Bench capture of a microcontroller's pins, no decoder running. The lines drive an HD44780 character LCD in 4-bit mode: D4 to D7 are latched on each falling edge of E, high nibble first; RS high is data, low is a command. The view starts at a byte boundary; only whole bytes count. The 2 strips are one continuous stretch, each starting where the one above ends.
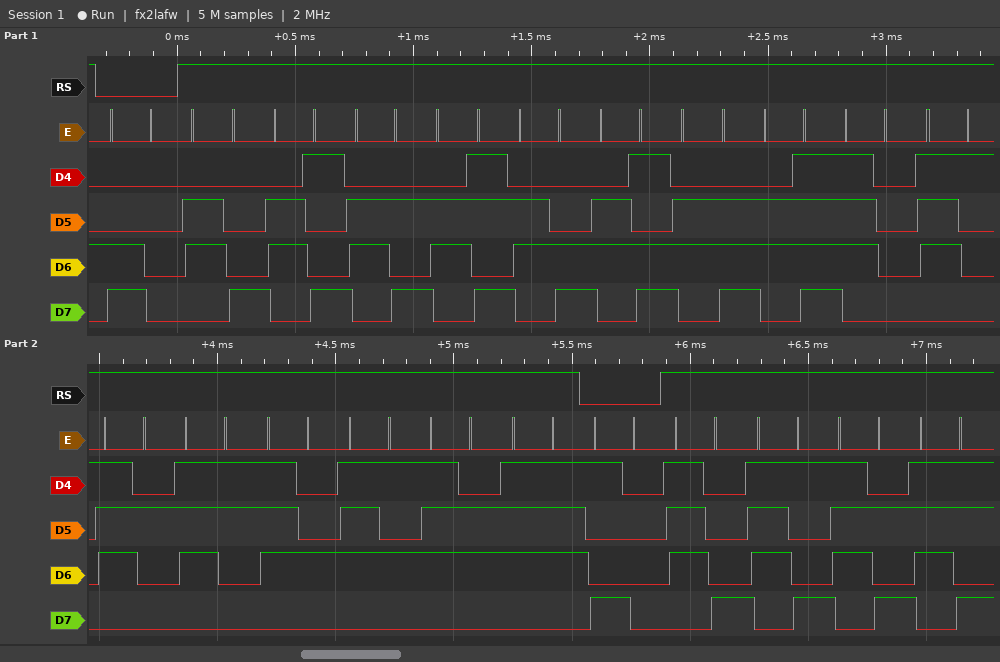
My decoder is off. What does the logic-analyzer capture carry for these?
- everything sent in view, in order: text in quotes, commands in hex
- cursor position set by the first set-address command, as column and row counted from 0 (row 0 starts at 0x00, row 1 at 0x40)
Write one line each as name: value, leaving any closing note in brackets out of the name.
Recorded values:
everything sent in view, in order: text in quotes, commands in hex: 0xC0 "hijklmnopqrstuvw" 0x90 "xyz{"
cursor position set by the first set-address command, as column and row counted from 0: column 0, row 1
